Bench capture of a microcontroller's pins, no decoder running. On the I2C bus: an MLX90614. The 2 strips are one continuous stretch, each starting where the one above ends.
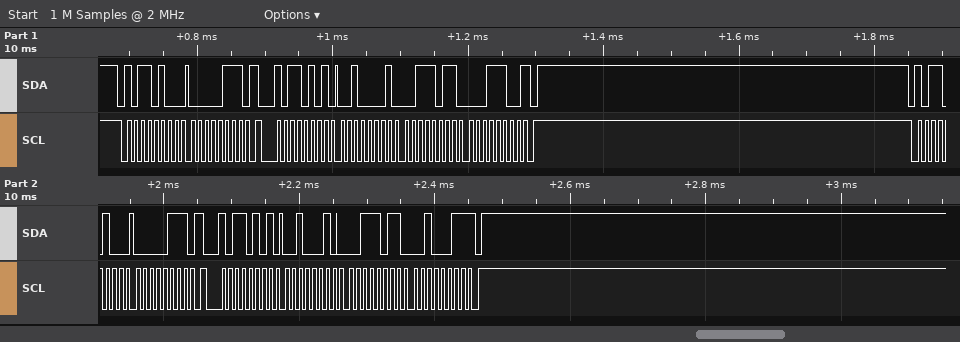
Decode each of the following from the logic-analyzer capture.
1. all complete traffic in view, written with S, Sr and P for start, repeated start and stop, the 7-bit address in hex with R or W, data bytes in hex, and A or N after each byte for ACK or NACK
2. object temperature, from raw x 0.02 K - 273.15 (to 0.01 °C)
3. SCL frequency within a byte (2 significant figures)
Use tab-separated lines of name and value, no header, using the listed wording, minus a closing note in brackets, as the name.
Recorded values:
all complete traffic in view, written with S, Sr and P for start, repeated start and stop, the 7-bit address in hex with R or W, data bytes in hex, and A or N after each byte for ACK or NACK	S 5AW A 07 A Sr 5AR A 21 A 3B A 1C N P S 5AW A 07 A Sr 5AR A 22 A 3B A 23 N P
object temperature, from raw x 0.02 K - 273.15	29.59 °C
SCL frequency within a byte	100 kHz
